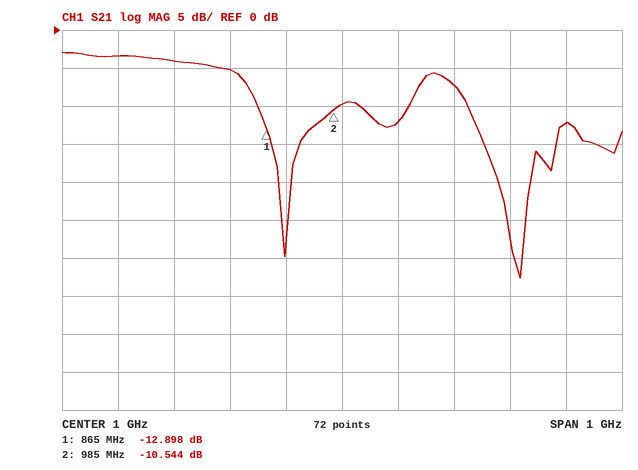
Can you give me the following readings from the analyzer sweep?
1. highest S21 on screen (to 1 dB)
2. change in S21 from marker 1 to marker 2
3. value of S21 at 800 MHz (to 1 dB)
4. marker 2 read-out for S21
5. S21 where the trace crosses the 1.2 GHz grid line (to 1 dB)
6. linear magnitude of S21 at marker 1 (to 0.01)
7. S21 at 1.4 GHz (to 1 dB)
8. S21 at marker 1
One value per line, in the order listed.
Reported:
-3 dB
2.354 dB
-5 dB
-10.544 dB
-7 dB
0.23
-12 dB
-12.898 dB
